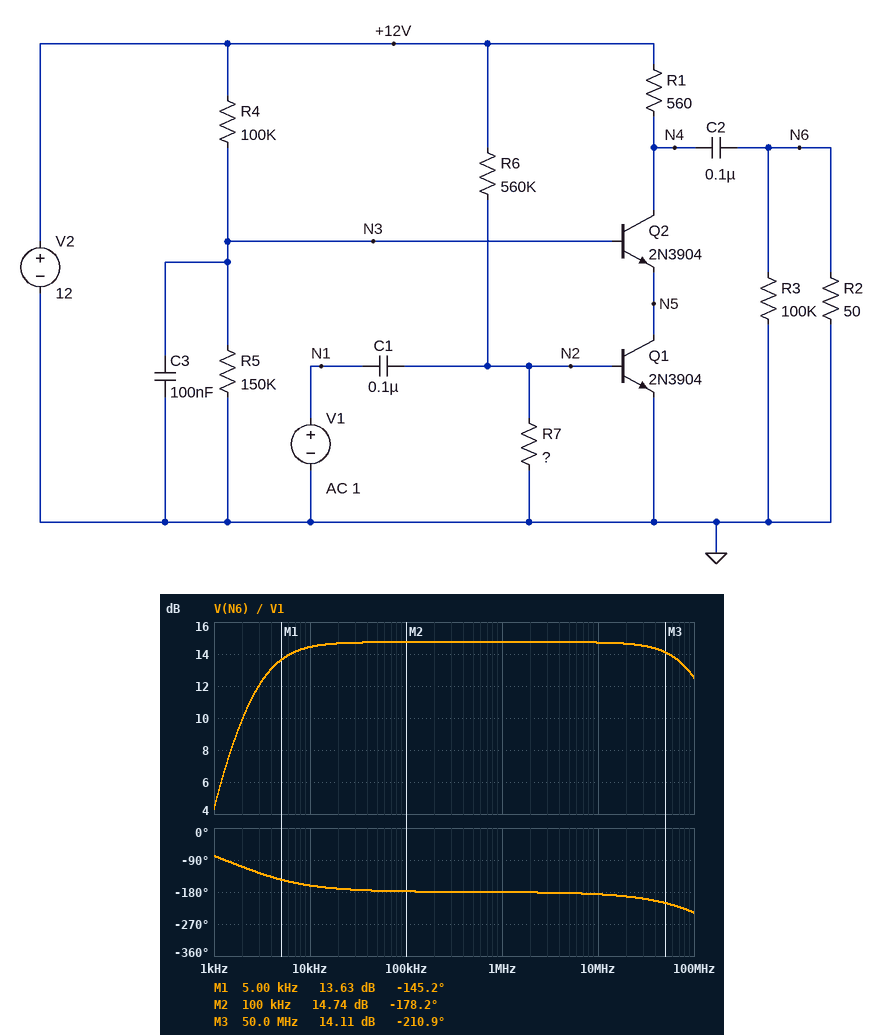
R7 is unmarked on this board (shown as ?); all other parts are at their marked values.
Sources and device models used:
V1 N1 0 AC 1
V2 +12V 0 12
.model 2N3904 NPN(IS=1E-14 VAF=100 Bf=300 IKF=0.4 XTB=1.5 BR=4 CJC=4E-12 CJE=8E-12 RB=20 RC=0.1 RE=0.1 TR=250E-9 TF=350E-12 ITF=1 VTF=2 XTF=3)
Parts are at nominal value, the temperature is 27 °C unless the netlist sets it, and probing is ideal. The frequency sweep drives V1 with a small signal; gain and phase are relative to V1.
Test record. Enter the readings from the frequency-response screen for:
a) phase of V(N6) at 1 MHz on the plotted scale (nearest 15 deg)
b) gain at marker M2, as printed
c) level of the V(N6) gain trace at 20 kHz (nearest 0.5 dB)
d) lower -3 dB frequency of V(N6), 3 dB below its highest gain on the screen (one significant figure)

-180 deg
14.74 dB
14.5 dB
3 kHz
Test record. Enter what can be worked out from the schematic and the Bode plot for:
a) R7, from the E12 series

68 kΩ
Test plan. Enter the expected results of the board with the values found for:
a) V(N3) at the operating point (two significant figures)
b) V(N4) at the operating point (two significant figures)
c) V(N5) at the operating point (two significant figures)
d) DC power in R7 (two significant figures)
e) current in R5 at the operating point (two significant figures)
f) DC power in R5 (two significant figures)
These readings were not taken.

6.6 V
10 V
5.9 V
6.9 µW
44 µA
290 µW
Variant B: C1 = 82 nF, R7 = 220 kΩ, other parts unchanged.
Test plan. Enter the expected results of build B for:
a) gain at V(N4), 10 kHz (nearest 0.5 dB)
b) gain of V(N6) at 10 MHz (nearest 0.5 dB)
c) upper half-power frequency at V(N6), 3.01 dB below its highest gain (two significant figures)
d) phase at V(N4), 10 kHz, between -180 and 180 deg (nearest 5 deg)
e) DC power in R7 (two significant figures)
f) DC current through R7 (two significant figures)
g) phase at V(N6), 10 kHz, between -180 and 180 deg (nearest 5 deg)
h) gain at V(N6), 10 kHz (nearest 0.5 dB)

29.0 dB
19.0 dB
89 MHz
130 deg
2.2 µW
3.2 µA
-160 deg
18.5 dB
